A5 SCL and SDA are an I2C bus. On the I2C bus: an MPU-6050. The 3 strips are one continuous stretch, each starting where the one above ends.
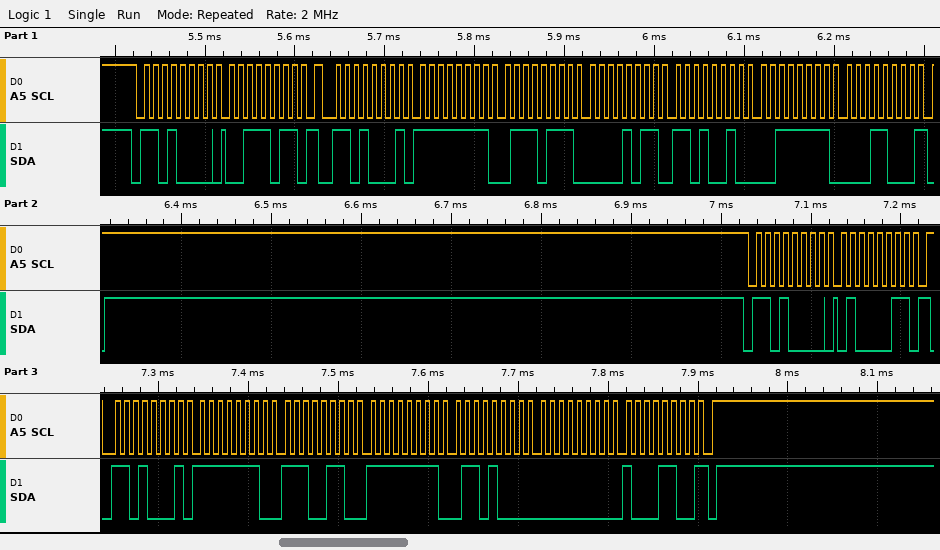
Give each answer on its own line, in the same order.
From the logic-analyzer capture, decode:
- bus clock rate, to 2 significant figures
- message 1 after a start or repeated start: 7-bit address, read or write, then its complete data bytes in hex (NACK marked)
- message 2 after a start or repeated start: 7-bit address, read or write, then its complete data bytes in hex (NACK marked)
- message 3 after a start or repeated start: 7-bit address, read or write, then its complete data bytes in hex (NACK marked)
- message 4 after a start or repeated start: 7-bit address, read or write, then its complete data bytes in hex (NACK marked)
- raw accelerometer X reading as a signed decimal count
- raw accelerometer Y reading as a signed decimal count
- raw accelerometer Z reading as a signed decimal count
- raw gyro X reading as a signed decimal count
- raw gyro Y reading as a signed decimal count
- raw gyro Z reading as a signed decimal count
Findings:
100 kHz
0x68 write: 3B
0x68 read: FF 77 0B D2 3F 18 NACK
0x68 write: 43
0x68 read: FE E6 FF 68 00 8C NACK
-137
3026
16152
-282
-152
140
